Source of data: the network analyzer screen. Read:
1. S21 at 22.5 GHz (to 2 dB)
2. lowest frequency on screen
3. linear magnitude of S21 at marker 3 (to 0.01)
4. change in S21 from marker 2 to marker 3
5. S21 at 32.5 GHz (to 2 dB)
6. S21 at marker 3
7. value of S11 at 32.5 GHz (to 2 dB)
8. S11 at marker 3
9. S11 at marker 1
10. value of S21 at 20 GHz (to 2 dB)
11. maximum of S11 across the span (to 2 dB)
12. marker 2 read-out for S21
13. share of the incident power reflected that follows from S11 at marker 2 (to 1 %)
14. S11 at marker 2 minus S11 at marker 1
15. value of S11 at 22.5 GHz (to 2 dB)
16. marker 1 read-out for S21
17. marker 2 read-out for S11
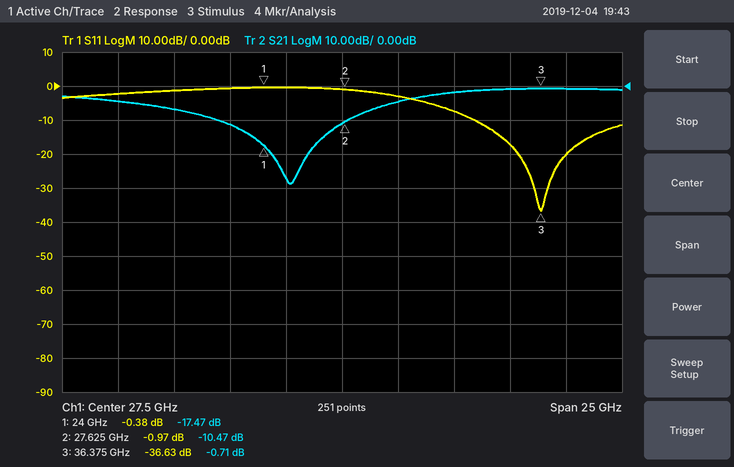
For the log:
-12 dB
15 GHz
0.92
9.76 dB
-2 dB
-0.71 dB
-8 dB
-36.63 dB
-0.38 dB
-6 dB
0 dB
-10.47 dB
80 %
-0.59 dB
0 dB
-17.47 dB
-0.97 dB
